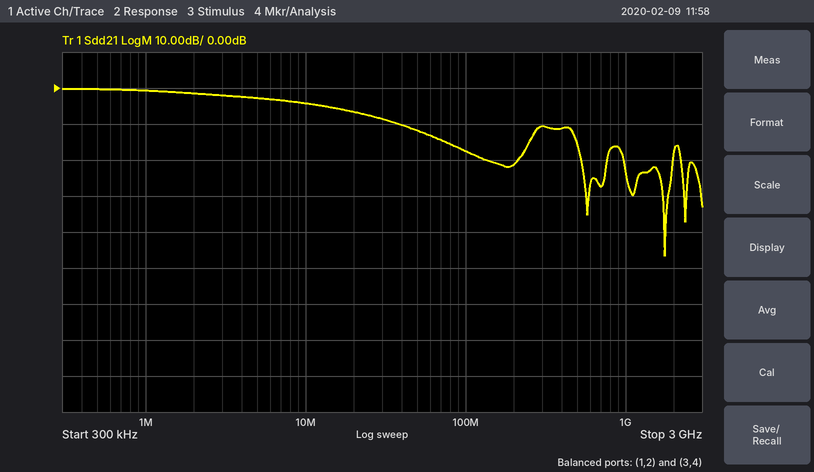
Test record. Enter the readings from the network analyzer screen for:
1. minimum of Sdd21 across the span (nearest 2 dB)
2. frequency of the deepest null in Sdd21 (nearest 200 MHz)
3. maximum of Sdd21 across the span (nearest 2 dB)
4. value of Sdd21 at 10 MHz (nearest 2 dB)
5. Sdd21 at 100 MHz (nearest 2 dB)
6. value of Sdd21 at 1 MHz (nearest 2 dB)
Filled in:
-46 dB
1.8 GHz
0 dB
-4 dB
-18 dB
0 dB
